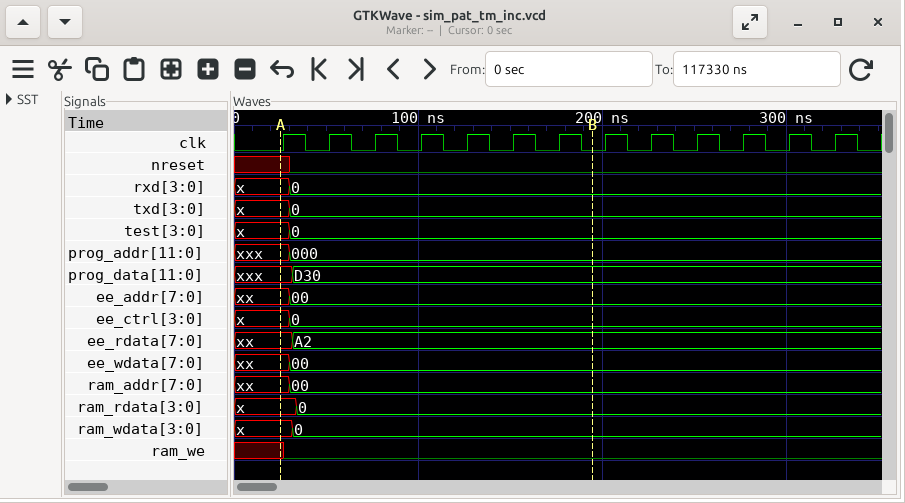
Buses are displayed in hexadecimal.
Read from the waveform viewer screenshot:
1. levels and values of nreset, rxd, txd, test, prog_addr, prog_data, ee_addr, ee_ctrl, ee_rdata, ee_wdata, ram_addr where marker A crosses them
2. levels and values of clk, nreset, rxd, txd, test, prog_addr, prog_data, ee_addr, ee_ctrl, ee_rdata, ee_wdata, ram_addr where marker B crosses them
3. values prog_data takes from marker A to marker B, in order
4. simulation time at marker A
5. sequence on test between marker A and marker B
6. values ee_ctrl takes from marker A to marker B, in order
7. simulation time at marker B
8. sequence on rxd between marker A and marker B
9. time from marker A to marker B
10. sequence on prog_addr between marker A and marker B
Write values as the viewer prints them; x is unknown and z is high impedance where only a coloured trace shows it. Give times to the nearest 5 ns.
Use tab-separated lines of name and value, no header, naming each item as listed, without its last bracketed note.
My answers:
levels and values of nreset, rxd, txd, test, prog_addr, prog_data, ee_addr, ee_ctrl, ee_rdata, ee_wdata, ram_addr where marker A crosses them	nreset=x, rxd=x, txd=x, test=x, prog_addr=xxx, prog_data=xxx, ee_addr=xx, ee_ctrl=x, ee_rdata=xx, ee_wdata=xx, ram_addr=xx
levels and values of clk, nreset, rxd, txd, test, prog_addr, prog_data, ee_addr, ee_ctrl, ee_rdata, ee_wdata, ram_addr where marker B crosses them	clk=0, nreset=0, rxd=0, txd=0, test=0, prog_addr=000, prog_data=D30, ee_addr=00, ee_ctrl=0, ee_rdata=A2, ee_wdata=00, ram_addr=00
values prog_data takes from marker A to marker B, in order	xxx, D30
simulation time at marker A	25 ns
sequence on test between marker A and marker B	x, 0
values ee_ctrl takes from marker A to marker B, in order	x, 0
simulation time at marker B	195 ns
sequence on rxd between marker A and marker B	x, 0
time from marker A to marker B	170 ns
sequence on prog_addr between marker A and marker B	xxx, 000
